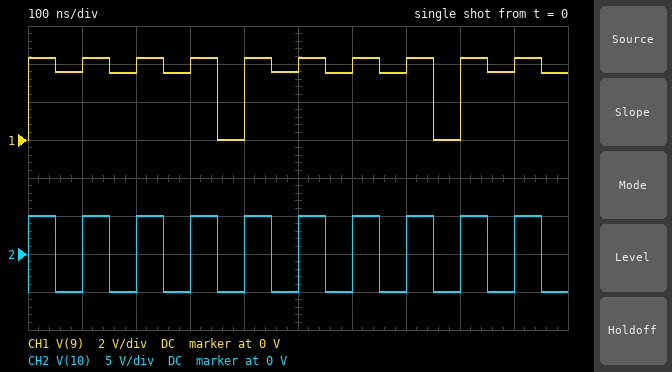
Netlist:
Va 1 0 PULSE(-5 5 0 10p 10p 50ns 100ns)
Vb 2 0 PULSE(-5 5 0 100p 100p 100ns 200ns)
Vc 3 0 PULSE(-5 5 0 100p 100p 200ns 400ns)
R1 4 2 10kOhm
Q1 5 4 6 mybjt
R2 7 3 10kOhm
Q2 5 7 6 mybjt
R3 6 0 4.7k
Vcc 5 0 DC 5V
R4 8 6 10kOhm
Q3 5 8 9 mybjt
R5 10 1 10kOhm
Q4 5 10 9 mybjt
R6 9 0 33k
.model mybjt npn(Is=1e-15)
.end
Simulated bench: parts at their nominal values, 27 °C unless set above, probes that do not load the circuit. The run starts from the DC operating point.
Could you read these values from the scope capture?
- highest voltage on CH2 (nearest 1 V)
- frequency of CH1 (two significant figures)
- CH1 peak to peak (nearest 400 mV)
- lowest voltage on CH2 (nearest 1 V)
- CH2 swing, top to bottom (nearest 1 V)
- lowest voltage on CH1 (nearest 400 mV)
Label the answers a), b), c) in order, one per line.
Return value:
a) 5 V
b) 2.5 MHz
c) 4.4 V
d) -5 V
e) 10 V
f) 0 V
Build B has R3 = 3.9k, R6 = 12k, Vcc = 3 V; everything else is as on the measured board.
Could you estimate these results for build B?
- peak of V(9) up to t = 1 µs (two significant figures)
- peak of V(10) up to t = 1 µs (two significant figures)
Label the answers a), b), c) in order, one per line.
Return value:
a) 3.0 V
b) 3.7 V
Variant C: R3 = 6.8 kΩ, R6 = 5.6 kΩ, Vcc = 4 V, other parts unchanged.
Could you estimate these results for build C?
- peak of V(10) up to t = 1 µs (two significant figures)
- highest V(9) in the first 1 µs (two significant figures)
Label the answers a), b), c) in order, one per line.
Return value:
a) 4.6 V
b) 3.9 V
